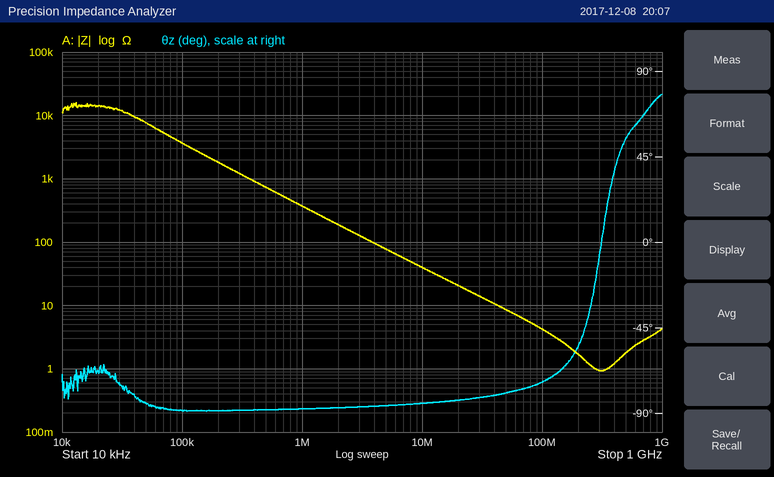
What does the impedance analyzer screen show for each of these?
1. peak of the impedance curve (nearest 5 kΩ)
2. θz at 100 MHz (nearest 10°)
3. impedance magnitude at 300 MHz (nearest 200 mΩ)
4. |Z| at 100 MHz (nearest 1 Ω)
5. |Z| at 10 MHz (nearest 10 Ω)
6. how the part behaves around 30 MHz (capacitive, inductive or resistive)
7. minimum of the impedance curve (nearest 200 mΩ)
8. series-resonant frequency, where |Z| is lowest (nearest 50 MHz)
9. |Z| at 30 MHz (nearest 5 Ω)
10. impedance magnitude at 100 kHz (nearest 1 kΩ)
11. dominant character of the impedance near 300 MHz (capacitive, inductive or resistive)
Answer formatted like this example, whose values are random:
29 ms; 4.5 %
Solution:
15 kΩ; -70°; 1.0 Ω; 4 Ω; 40 Ω; capacitive; 1.0 Ω; 300 MHz; 15 Ω; 4 kΩ; resistive
